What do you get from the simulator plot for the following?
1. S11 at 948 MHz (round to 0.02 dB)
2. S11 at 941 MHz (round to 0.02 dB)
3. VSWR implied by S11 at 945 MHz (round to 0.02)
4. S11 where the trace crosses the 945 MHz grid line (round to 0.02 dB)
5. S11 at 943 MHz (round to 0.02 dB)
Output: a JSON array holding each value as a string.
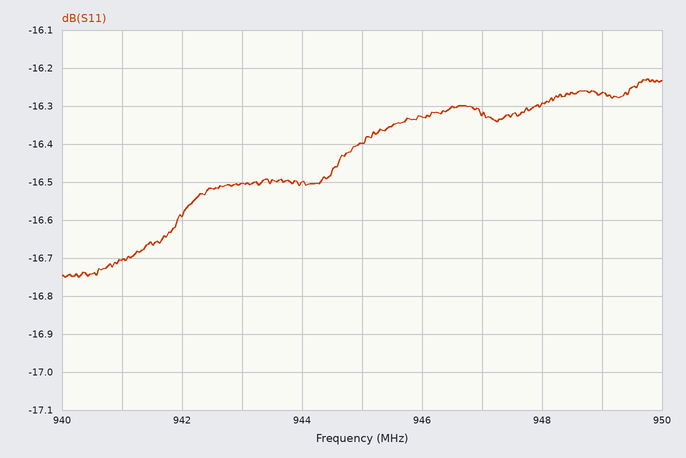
["-16.30 dB", "-16.70 dB", "1.36", "-16.40 dB", "-16.50 dB"]
